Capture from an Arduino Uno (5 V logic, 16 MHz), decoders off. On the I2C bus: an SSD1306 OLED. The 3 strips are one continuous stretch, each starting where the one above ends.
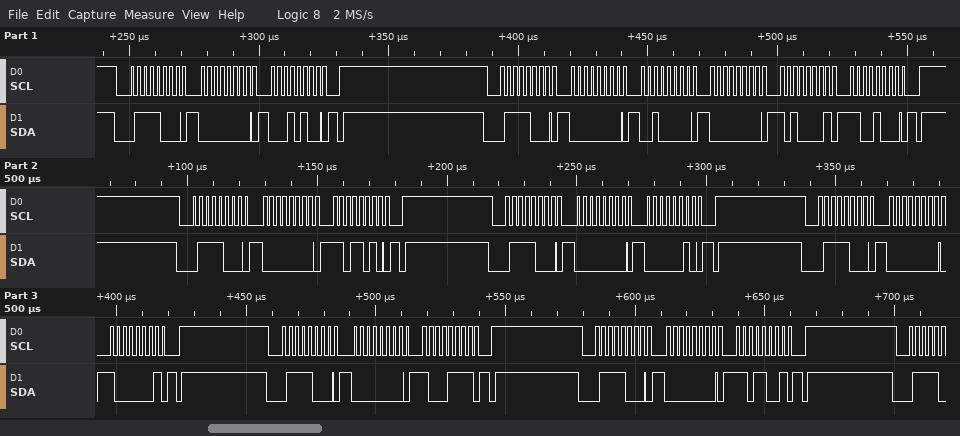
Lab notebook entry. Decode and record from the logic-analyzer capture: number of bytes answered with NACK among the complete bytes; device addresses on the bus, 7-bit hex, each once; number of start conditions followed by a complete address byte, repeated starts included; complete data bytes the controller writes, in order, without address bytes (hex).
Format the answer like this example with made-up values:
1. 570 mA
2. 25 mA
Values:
1. 0
2. 0x3C
3. 7
4. 00 14 00 20 00 A1 C8 00 DA 00 02 00 81 00 8F 00 D9
